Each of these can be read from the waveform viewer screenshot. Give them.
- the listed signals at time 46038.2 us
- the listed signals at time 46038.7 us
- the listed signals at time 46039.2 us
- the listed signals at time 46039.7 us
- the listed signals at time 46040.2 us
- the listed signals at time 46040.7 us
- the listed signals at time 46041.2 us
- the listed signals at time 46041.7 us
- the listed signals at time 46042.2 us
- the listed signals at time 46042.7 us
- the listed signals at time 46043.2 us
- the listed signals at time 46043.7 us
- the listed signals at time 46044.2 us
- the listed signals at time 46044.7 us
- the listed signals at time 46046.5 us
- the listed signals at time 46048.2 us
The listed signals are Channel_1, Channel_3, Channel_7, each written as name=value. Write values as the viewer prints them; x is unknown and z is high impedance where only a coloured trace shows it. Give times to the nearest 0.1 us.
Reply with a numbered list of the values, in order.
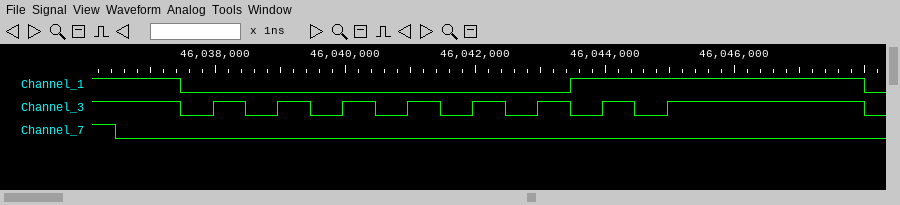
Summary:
1. Channel_1=0, Channel_3=1, Channel_7=0
2. Channel_1=0, Channel_3=0, Channel_7=0
3. Channel_1=0, Channel_3=1, Channel_7=0
4. Channel_1=0, Channel_3=0, Channel_7=0
5. Channel_1=0, Channel_3=1, Channel_7=0
6. Channel_1=0, Channel_3=0, Channel_7=0
7. Channel_1=0, Channel_3=1, Channel_7=0
8. Channel_1=0, Channel_3=0, Channel_7=0
9. Channel_1=0, Channel_3=1, Channel_7=0
10. Channel_1=0, Channel_3=0, Channel_7=0
11. Channel_1=0, Channel_3=1, Channel_7=0
12. Channel_1=1, Channel_3=0, Channel_7=0
13. Channel_1=1, Channel_3=1, Channel_7=0
14. Channel_1=1, Channel_3=0, Channel_7=0
15. Channel_1=1, Channel_3=1, Channel_7=0
16. Channel_1=0, Channel_3=0, Channel_7=0
